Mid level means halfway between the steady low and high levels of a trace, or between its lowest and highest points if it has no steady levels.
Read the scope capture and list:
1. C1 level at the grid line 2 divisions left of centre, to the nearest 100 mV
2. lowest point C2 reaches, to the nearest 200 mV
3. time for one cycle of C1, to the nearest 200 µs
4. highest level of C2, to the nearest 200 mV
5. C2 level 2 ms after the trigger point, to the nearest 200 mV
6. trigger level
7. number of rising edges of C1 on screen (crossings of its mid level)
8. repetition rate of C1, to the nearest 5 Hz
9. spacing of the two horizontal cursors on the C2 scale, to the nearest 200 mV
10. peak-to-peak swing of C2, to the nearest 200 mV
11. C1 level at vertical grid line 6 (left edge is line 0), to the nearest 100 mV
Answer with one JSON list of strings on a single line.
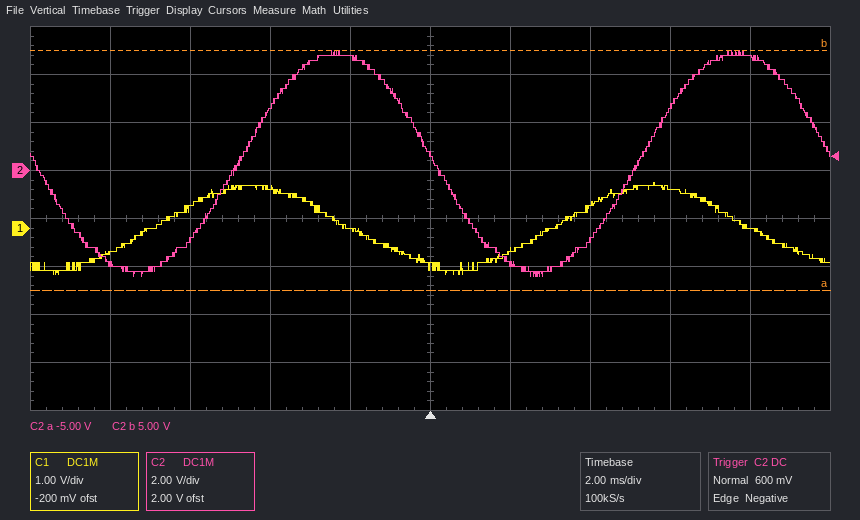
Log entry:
["800 mV", "-4.4 V", "10.0 ms", "5.0 V", "-3.8 V", "600 mV", "2", "100 Hz", "10.0 V", "9.4 V", "-500 mV"]
